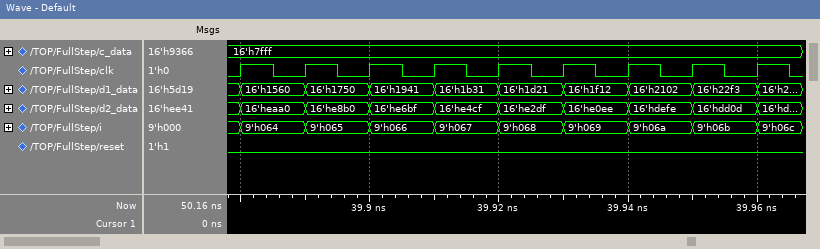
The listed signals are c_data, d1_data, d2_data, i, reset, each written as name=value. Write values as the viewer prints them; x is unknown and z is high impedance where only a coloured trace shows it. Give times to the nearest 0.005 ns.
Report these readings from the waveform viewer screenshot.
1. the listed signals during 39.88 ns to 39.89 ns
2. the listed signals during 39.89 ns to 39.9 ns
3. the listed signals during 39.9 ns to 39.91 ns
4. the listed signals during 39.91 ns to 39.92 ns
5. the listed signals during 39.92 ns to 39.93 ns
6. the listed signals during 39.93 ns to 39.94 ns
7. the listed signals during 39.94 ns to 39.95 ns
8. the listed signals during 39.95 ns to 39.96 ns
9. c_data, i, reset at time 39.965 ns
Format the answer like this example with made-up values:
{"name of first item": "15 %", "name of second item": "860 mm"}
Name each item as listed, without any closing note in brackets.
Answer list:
{"the listed signals during 39.88 ns to 39.89 ns": "c_data=16'h7fff, d1_data=16'h1560, d2_data=16'heaa0, i=9'h064, reset=0", "the listed signals during 39.89 ns to 39.9 ns": "c_data=16'h7fff, d1_data=16'h1750, d2_data=16'he8b0, i=9'h065, reset=0", "the listed signals during 39.9 ns to 39.91 ns": "c_data=16'h7fff, d1_data=16'h1941, d2_data=16'he6bf, i=9'h066, reset=0", "the listed signals during 39.91 ns to 39.92 ns": "c_data=16'h7fff, d1_data=16'h1b31, d2_data=16'he4cf, i=9'h067, reset=0", "the listed signals during 39.92 ns to 39.93 ns": "c_data=16'h7fff, d1_data=16'h1d21, d2_data=16'he2df, i=9'h068, reset=0", "the listed signals during 39.93 ns to 39.94 ns": "c_data=16'h7fff, d1_data=16'h1f12, d2_data=16'he0ee, i=9'h069, reset=0", "the listed signals during 39.94 ns to 39.95 ns": "c_data=16'h7fff, d1_data=16'h2102, d2_data=16'hdefe, i=9'h06a, reset=0", "the listed signals during 39.95 ns to 39.96 ns": "c_data=16'h7fff, d1_data=16'h22f3, d2_data=16'hdd0d, i=9'h06b, reset=0", "c_data, i, reset at time 39.965 ns": "c_data=16'h7fff, i=9'h06c, reset=0"}
